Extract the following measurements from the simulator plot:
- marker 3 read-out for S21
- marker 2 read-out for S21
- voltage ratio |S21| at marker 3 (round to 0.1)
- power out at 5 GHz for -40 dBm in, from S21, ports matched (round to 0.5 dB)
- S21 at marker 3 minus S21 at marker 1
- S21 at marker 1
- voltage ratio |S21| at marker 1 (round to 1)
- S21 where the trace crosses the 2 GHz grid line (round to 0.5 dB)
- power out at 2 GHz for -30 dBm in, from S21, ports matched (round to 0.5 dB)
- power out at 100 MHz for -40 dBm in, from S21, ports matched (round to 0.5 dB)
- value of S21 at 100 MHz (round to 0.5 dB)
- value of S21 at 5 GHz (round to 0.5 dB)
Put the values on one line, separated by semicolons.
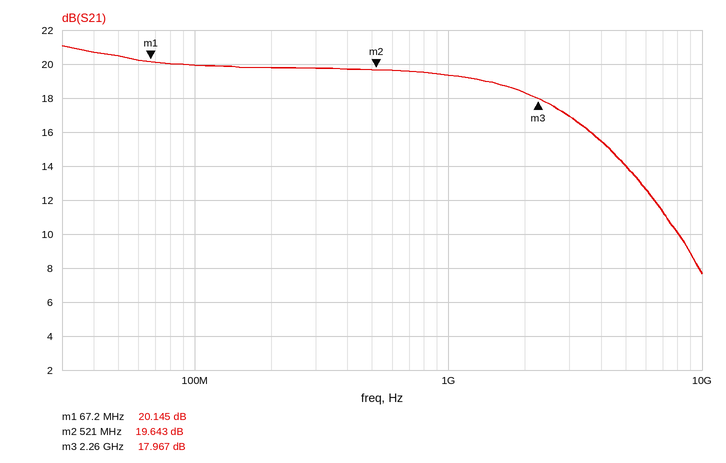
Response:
17.967 dB; 19.643 dB; 7.9; -26.0 dBm; -2.178 dB; 20.145 dB; 10; 18.5 dB; -11.5 dBm; -20.0 dBm; 20.0 dB; 14.0 dB
